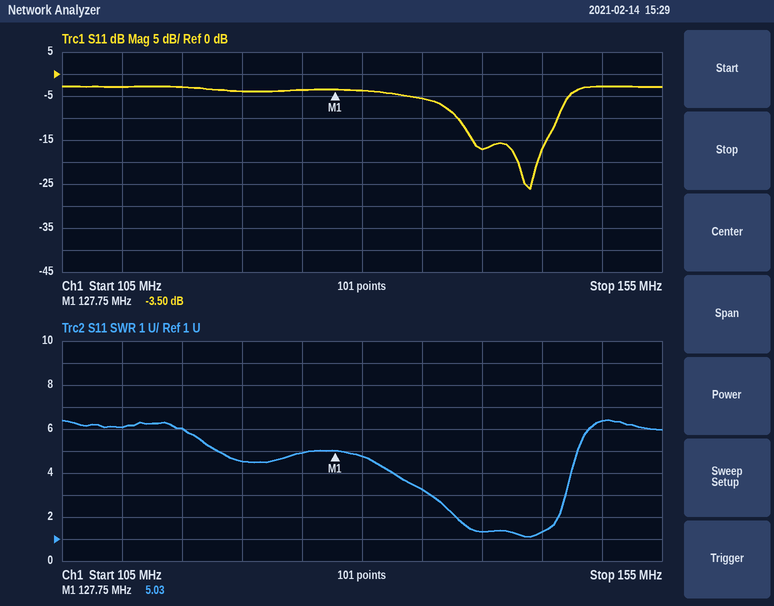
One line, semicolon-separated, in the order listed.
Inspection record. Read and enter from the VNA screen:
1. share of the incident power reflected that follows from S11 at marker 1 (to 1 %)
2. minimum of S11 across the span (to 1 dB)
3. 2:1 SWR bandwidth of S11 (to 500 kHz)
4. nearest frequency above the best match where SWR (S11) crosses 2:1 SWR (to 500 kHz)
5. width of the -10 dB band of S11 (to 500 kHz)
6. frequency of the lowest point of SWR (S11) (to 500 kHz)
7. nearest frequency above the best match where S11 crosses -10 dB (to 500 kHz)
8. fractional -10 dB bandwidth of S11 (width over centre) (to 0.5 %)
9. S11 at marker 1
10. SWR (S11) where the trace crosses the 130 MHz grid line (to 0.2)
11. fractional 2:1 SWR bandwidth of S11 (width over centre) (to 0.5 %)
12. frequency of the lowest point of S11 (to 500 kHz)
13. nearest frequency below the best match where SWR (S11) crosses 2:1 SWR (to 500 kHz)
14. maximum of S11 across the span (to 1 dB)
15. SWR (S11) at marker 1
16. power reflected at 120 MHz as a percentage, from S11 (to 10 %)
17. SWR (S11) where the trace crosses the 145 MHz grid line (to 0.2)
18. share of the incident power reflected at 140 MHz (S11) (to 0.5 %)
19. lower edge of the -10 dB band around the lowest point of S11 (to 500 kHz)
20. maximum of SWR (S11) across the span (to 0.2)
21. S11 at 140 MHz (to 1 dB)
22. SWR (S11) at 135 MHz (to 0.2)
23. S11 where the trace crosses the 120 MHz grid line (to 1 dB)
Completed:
45 %; -26 dB; 8.5 MHz; 146.5 MHz; 8.5 MHz; 144.0 MHz; 146.5 MHz; 6.0 %; -3.50 dB; 4.8; 6.0 %; 144.0 MHz; 138.0 MHz; -3 dB; 5.03; 40 %; 1.4; 2.0 %; 138.0 MHz; 6.4; -17 dB; 3.2; -4 dB
